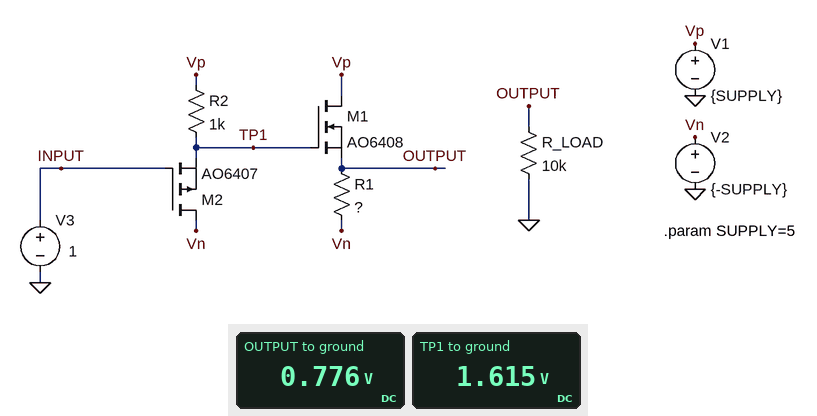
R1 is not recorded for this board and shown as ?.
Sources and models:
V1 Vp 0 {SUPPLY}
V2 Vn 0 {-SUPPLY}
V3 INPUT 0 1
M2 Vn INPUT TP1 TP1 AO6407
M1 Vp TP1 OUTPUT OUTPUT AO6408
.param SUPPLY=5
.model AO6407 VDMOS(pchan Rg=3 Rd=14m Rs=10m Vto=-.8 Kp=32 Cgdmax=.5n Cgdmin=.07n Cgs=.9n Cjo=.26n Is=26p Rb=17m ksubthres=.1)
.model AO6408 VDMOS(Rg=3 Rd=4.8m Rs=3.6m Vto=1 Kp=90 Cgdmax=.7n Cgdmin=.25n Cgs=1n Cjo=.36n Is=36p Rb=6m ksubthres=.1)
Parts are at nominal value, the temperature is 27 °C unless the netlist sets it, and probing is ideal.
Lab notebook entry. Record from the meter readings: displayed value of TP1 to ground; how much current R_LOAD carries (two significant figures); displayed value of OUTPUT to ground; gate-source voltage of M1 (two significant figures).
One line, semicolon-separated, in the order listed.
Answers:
1.615 V; 78 µA; 0.776 V; 840 mV
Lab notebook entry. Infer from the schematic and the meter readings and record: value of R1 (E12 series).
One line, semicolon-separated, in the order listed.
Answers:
390 Ω
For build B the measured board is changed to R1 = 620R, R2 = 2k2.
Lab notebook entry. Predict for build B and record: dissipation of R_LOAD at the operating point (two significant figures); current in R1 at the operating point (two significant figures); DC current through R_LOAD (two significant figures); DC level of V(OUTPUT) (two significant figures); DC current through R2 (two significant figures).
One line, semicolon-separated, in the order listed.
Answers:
58 µW; 9.3 mA; 76 µA; 760 mV; 1.6 mA
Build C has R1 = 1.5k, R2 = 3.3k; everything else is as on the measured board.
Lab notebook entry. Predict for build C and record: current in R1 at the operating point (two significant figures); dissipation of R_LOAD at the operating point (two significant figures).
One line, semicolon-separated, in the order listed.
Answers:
3.9 mA; 62 µW
